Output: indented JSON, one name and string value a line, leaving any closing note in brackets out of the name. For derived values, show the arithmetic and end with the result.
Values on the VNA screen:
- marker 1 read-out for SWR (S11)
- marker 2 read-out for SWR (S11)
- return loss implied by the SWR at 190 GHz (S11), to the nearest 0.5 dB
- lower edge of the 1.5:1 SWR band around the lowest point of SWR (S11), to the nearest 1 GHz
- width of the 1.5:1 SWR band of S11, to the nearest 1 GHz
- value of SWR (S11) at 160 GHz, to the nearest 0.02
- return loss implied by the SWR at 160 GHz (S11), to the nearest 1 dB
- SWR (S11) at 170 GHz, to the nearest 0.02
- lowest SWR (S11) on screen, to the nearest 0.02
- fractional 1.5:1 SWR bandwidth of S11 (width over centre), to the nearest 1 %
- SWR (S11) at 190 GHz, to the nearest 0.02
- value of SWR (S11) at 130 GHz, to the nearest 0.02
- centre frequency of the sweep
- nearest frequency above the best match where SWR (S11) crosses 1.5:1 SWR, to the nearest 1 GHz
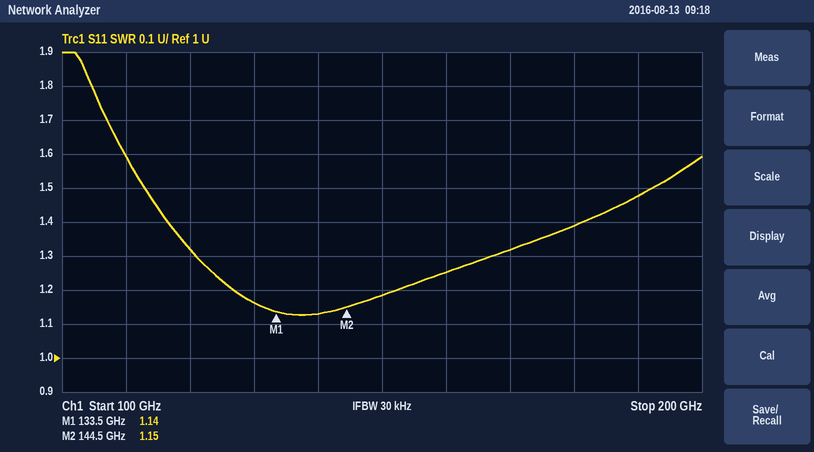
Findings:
{
  "marker 1 read-out for SWR": "1.14",
  "marker 2 read-out for SWR": "1.15",
  "return loss implied by the SWR at 190 GHz (S11), to the nearest 0.5 dB": "−20 log10((1.48 − 1)/(1.48 + 1)) ≈ 14.3 dB, so 14.5 dB to the nearest 0.5 dB",
  "lower edge of the 1.5:1 SWR band around the lowest point of SWR (S11), to the nearest 1 GHz": "113 GHz",
  "width of the 1.5:1 SWR band of S11, to the nearest 1 GHz": "192 GHz − 113 GHz = 79 GHz",
  "value of SWR (S11) at 160 GHz, to the nearest 0.02": "1.26",
  "return loss implied by the SWR at 160 GHz (S11), to the nearest 1 dB": "−20 log10((1.26 − 1)/(1.26 + 1)) ≈ 19 dB",
  "SWR (S11) at 170 GHz, to the nearest 0.02": "1.32",
  "lowest SWR (S11) on screen, to the nearest 0.02": "1.12",
  "fractional 1.5:1 SWR bandwidth of S11 (width over centre), to the nearest 1 %": "79 GHz / 152.5 GHz ≈ 52 %",
  "SWR (S11) at 190 GHz, to the nearest 0.02": "1.48",
  "value of SWR (S11) at 130 GHz, to the nearest 0.02": "1.16",
  "centre frequency of the sweep": "150 GHz",
  "nearest frequency above the best match where SWR (S11) crosses 1.5:1 SWR, to the nearest 1 GHz": "192 GHz"
}
